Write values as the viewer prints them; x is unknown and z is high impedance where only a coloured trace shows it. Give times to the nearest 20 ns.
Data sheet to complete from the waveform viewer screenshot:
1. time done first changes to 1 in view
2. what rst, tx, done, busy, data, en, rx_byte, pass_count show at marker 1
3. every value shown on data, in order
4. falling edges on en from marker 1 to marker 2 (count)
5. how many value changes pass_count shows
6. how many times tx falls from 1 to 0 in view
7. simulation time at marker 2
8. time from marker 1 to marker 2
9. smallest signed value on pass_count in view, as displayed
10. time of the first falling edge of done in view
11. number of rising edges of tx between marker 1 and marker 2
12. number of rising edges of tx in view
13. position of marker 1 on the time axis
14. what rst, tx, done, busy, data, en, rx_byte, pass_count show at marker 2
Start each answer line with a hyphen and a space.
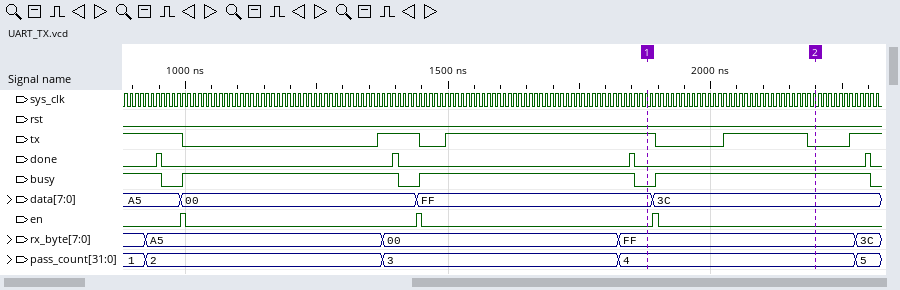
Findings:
- 940 ns
- rst=0, tx=1, done=0, busy=0, data=FF, en=0, rx_byte=FF, pass_count=4
- A5, 00, FF, 3C
- 1
- 4
- 4
- 2200 ns
- 320 ns
- 1
- 960 ns
- 1
- 4
- 1880 ns
- rst=0, tx=0, done=0, busy=1, data=3C, en=0, rx_byte=FF, pass_count=4
